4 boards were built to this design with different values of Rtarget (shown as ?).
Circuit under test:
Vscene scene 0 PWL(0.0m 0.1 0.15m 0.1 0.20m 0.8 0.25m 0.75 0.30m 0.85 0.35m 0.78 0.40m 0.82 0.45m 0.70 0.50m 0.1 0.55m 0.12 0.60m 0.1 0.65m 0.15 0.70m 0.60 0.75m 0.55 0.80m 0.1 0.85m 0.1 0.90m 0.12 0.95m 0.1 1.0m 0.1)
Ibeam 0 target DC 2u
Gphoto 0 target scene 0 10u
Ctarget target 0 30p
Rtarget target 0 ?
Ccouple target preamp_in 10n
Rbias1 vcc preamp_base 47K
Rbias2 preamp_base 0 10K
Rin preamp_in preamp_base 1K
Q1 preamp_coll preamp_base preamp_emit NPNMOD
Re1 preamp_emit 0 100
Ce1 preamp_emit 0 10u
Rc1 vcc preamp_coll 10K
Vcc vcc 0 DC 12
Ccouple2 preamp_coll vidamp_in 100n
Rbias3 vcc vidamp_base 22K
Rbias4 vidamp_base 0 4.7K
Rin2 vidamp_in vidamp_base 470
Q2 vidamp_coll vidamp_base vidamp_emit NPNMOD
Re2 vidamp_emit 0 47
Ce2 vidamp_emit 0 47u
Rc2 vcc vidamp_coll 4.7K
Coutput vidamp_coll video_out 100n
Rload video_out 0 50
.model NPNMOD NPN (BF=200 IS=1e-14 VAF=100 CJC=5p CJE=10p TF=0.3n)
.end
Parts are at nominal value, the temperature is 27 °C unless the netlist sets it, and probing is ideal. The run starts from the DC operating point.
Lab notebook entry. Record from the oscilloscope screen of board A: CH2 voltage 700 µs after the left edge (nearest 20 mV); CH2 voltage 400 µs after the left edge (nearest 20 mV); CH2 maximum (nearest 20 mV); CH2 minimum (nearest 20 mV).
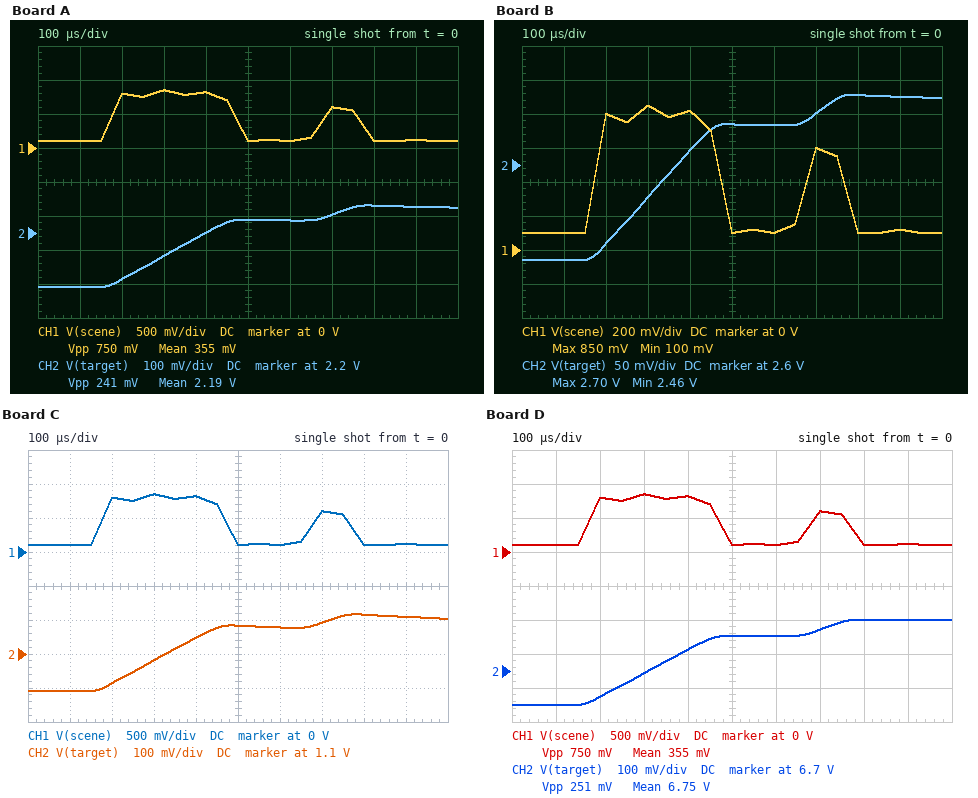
2.26 V
2.20 V
2.28 V
2.04 V
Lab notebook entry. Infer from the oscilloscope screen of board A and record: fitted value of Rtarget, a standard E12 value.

680 kΩ
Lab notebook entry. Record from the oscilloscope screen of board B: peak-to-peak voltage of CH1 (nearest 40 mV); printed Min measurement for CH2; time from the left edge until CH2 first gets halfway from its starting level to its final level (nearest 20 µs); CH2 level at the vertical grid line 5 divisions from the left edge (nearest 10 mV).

760 mV
2.46 V
340 µs
2.66 V
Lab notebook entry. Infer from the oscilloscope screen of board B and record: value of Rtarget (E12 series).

820 kΩ
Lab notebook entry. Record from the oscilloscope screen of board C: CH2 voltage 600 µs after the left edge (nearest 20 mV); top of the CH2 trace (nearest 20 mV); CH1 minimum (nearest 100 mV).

1.18 V
1.22 V
100 mV
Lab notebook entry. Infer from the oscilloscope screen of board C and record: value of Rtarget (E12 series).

330 kΩ
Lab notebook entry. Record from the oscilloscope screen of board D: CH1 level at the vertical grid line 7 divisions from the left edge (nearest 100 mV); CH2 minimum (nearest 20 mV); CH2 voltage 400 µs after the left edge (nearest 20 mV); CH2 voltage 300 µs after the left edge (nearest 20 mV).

600 mV
6.60 V
6.76 V
6.70 V
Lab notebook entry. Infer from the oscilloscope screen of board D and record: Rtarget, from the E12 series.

2.2 MΩ
